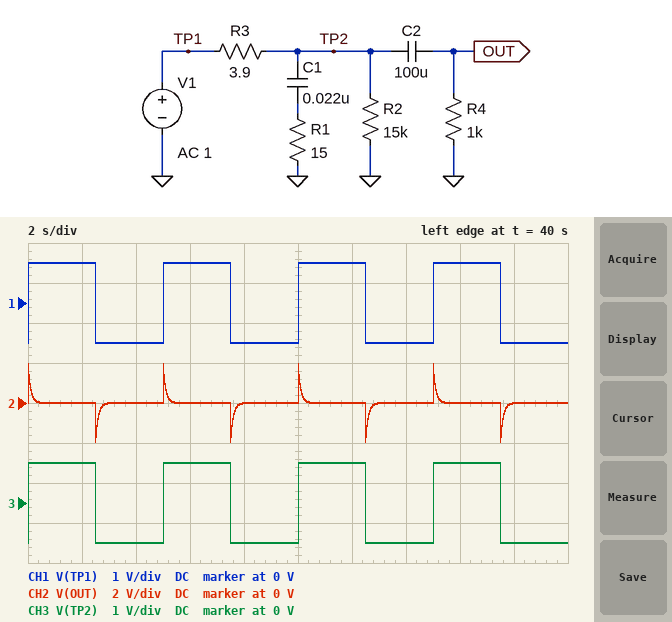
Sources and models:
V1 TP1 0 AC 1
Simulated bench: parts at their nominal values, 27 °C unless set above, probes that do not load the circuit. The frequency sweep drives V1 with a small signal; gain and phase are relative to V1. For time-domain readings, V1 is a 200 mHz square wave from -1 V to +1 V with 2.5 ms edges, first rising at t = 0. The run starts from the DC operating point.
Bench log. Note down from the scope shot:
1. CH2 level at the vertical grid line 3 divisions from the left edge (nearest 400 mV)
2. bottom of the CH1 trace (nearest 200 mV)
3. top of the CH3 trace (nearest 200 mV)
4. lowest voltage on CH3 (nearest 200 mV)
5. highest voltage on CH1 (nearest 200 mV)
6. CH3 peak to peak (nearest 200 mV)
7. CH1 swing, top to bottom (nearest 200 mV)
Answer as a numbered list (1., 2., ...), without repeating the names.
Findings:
1. 0 V
2. -1.0 V
3. 1.0 V
4. -1.0 V
5. 1.0 V
6. 2.0 V
7. 2.0 V
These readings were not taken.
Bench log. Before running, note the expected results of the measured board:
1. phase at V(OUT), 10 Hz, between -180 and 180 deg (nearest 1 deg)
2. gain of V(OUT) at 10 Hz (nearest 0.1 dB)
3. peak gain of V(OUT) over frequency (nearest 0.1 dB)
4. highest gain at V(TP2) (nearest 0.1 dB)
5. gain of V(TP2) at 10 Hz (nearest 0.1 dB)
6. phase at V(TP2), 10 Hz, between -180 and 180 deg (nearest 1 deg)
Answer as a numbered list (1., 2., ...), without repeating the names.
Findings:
1. 9 deg
2. -0.1 dB
3. 0 dB
4. 0 dB
5. 0 dB
6. 0 deg
